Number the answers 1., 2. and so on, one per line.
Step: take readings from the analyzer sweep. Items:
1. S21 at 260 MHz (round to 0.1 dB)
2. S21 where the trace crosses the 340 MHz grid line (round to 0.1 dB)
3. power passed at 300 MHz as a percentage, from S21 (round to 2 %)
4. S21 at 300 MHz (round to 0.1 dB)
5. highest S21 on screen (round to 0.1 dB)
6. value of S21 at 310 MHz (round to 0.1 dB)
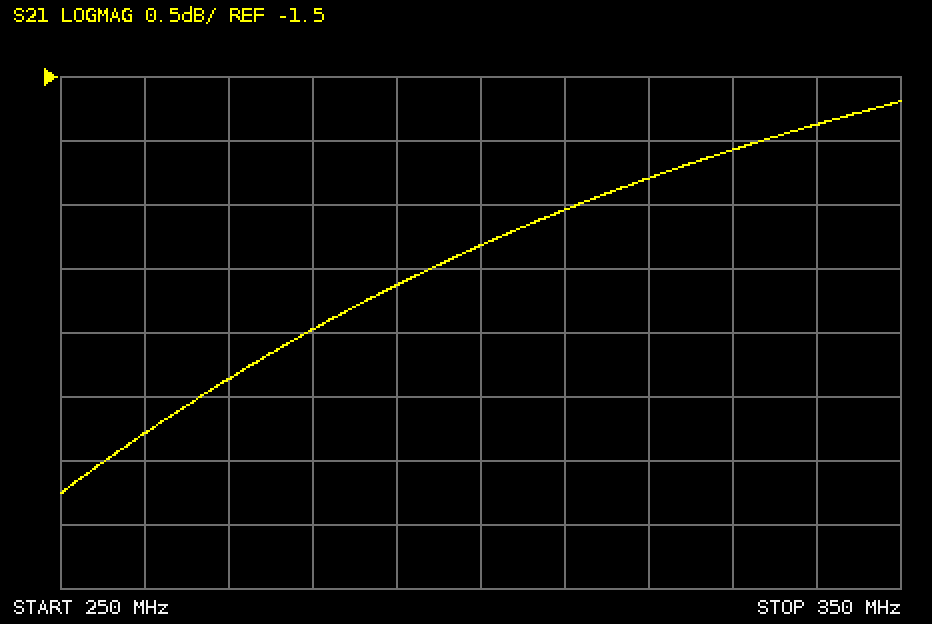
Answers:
1. -4.3 dB
2. -1.9 dB
3. 52 %
4. -2.8 dB
5. -1.7 dB
6. -2.5 dB
